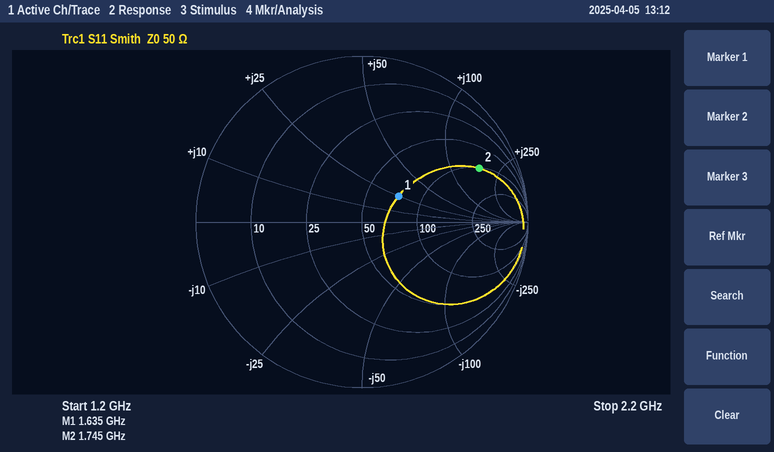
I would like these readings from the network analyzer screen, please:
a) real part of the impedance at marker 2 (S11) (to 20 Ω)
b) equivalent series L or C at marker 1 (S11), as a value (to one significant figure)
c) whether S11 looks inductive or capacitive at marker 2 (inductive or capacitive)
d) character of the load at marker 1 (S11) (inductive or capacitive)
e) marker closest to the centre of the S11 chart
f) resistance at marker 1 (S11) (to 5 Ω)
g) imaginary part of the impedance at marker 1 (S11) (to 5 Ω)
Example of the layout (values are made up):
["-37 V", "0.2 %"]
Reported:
["100 Ω", "2 nH", "inductive", "inductive", "marker 1", "75 Ω", "+25 Ω"]
